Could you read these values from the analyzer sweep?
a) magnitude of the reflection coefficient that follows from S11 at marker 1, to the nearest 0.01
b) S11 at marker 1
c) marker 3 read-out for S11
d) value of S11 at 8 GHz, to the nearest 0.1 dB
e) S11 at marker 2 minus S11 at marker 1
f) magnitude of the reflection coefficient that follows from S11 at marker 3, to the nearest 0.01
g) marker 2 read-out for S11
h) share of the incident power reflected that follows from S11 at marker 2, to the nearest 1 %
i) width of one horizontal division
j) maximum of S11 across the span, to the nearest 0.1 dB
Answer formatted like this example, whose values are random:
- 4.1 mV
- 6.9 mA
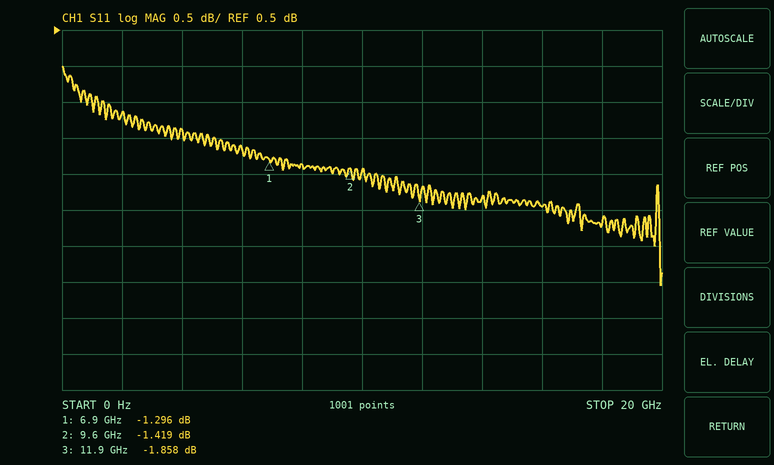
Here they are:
- 0.86
- -1.296 dB
- -1.858 dB
- -1.4 dB
- -0.123 dB
- 0.81
- -1.419 dB
- 72 %
- 2 GHz
- 0.0 dB
